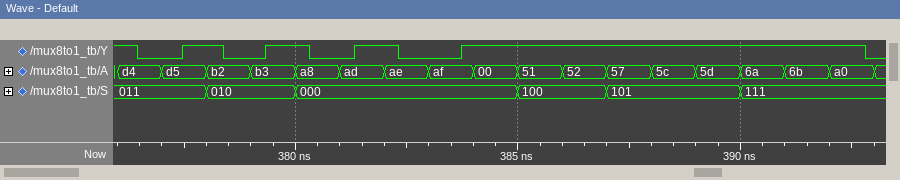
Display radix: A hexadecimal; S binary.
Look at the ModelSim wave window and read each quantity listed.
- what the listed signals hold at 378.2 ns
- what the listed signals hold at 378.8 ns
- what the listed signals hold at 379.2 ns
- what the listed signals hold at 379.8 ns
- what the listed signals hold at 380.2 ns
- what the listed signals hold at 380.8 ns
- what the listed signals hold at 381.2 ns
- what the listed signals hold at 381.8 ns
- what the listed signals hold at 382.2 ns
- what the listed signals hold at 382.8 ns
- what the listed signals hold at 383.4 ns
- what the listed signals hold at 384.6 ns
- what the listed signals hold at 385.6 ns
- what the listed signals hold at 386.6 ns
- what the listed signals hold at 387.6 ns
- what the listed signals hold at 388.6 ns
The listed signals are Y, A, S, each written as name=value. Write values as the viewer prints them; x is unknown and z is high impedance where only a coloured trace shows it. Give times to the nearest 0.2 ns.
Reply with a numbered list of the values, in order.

1. Y=1, A=b2, S=010
2. Y=0, A=b2, S=010
3. Y=0, A=b3, S=010
4. Y=1, A=b3, S=010
5. Y=1, A=a8, S=000
6. Y=0, A=a8, S=000
7. Y=0, A=ad, S=000
8. Y=1, A=ad, S=000
9. Y=1, A=ae, S=000
10. Y=0, A=ae, S=000
11. Y=0, A=af, S=000
12. Y=1, A=00, S=000
13. Y=1, A=51, S=100
14. Y=1, A=52, S=100
15. Y=1, A=57, S=101
16. Y=1, A=5c, S=101
